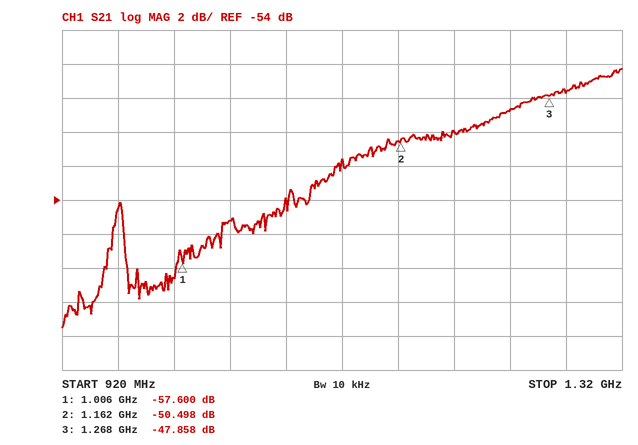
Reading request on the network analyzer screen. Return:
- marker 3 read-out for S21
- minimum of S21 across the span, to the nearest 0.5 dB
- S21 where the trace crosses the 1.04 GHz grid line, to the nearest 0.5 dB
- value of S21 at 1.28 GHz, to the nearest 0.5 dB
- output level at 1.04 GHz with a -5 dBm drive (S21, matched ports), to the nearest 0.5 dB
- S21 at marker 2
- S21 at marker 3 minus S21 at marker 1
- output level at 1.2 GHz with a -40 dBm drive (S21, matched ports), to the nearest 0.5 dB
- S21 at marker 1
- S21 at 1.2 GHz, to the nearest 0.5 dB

-47.858 dB
-61.5 dB
-55.0 dB
-47.5 dB
-60.0 dBm
-50.498 dB
9.742 dB
-90.0 dBm
-57.600 dB
-50.0 dB
